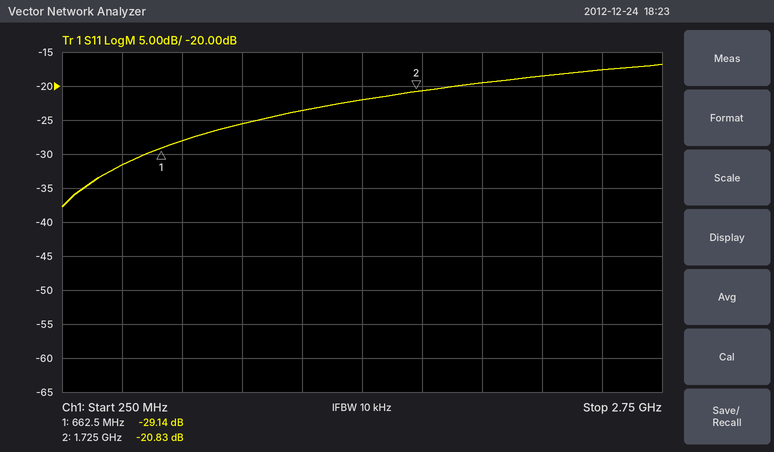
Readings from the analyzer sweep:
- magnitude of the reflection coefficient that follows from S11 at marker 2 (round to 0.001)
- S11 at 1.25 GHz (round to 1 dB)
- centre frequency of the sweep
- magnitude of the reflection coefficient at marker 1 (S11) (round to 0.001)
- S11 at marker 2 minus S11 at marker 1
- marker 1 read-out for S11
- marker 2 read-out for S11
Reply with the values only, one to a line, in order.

0.091
-24 dB
1.5 GHz
0.035
8.31 dB
-29.14 dB
-20.83 dB
